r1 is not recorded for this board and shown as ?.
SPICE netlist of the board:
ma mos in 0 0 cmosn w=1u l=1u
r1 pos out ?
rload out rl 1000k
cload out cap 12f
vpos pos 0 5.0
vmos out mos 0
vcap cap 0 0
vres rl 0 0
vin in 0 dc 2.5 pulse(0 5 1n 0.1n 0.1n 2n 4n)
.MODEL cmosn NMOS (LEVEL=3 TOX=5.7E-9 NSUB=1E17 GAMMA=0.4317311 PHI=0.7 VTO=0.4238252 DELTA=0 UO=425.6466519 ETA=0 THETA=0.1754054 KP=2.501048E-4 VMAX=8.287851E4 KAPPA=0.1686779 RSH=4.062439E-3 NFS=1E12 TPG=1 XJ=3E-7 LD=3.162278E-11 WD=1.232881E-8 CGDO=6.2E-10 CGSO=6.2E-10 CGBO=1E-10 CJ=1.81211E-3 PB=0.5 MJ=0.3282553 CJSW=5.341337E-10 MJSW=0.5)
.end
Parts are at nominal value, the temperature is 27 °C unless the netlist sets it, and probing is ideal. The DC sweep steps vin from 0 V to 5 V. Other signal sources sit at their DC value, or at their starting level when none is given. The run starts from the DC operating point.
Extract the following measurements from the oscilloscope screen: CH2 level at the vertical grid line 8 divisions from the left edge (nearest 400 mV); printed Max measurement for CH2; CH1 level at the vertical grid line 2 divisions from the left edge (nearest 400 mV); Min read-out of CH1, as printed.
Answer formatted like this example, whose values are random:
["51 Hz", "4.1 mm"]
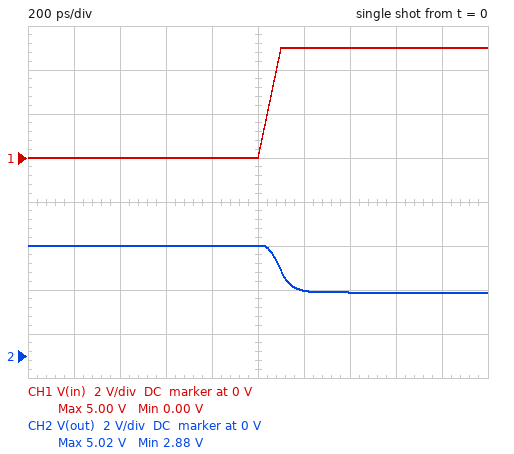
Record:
["2.8 V", "5.02 V", "0 V", "0.00 V"]
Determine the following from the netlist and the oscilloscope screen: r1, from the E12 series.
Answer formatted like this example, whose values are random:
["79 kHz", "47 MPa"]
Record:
["3.3 kΩ"]
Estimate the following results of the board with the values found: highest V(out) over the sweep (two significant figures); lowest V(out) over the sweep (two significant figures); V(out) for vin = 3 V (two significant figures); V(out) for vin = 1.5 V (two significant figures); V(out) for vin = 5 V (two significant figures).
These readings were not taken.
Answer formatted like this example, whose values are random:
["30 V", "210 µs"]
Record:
["5.0 V", "2.9 V", "4.0 V", "4.7 V", "2.9 V"]
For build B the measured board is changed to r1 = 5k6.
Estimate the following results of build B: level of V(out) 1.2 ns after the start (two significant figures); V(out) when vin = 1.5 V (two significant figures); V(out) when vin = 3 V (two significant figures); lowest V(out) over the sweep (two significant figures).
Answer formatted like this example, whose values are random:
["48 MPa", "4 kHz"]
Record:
["2.0 V", "4.5 V", "3.3 V", "1.8 V"]
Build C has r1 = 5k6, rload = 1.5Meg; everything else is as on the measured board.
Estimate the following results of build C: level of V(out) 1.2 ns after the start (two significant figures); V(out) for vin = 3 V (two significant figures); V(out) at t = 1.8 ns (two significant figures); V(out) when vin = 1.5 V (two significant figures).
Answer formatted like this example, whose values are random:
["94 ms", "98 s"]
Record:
["2.0 V", "3.3 V", "1.8 V", "4.5 V"]
